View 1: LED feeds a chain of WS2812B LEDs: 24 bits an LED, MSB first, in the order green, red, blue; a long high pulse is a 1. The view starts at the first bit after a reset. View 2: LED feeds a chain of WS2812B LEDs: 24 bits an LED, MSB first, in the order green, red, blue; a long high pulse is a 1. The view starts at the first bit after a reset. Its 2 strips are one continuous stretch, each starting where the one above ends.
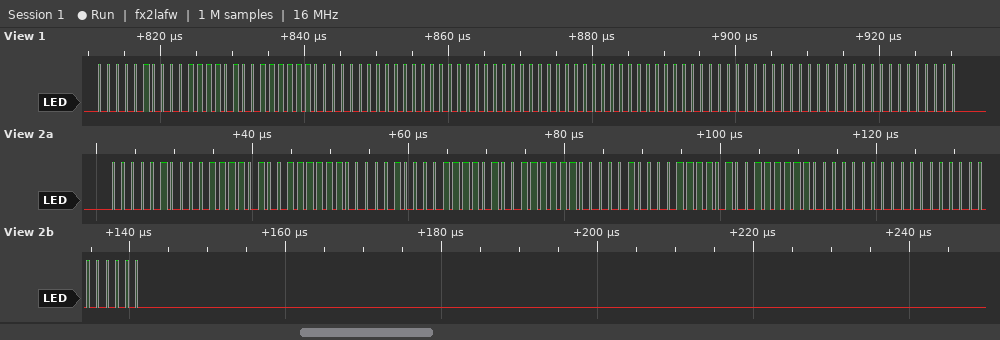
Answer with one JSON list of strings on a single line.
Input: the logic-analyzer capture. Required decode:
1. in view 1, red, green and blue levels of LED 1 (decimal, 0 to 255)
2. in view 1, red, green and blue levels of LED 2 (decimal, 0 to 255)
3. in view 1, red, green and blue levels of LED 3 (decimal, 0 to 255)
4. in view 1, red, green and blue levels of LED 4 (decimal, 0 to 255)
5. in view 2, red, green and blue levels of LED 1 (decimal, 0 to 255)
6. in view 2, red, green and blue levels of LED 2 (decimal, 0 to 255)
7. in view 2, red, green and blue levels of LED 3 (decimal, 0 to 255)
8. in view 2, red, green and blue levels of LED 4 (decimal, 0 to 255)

["61, 4, 63", "0, 0, 0", "0, 0, 0", "0, 0, 0", "61, 4, 63", "61, 4, 63", "61, 4, 63", "0, 0, 0"]
